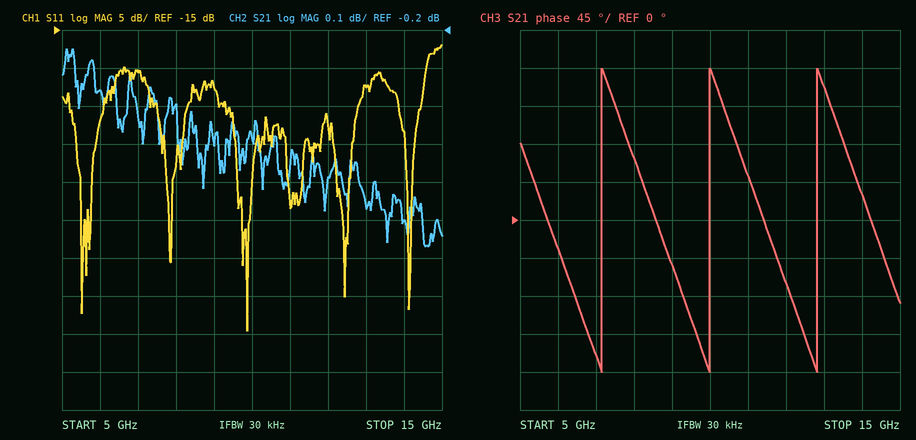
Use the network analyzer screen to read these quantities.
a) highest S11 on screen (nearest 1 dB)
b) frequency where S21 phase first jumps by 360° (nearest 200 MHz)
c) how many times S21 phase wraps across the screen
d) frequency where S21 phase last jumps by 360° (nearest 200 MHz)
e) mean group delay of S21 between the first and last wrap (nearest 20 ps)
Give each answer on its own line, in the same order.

-17 dB
7.2 GHz
3
12.8 GHz
360 ps
